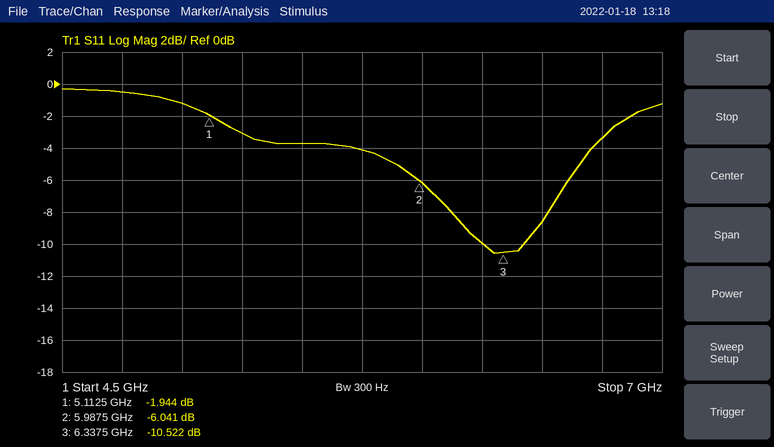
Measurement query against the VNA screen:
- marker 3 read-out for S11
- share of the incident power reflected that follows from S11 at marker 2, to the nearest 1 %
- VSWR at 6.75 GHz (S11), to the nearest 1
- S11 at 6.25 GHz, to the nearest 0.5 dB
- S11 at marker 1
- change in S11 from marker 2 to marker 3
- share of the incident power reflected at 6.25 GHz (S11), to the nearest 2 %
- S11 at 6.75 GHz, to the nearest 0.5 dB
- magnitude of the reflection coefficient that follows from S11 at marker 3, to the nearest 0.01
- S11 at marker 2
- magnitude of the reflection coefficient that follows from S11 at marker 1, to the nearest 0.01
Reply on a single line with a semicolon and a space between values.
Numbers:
-10.522 dB; 25 %; 5; -10.0 dB; -1.944 dB; -4.481 dB; 10 %; -3.5 dB; 0.30; -6.041 dB; 0.80
